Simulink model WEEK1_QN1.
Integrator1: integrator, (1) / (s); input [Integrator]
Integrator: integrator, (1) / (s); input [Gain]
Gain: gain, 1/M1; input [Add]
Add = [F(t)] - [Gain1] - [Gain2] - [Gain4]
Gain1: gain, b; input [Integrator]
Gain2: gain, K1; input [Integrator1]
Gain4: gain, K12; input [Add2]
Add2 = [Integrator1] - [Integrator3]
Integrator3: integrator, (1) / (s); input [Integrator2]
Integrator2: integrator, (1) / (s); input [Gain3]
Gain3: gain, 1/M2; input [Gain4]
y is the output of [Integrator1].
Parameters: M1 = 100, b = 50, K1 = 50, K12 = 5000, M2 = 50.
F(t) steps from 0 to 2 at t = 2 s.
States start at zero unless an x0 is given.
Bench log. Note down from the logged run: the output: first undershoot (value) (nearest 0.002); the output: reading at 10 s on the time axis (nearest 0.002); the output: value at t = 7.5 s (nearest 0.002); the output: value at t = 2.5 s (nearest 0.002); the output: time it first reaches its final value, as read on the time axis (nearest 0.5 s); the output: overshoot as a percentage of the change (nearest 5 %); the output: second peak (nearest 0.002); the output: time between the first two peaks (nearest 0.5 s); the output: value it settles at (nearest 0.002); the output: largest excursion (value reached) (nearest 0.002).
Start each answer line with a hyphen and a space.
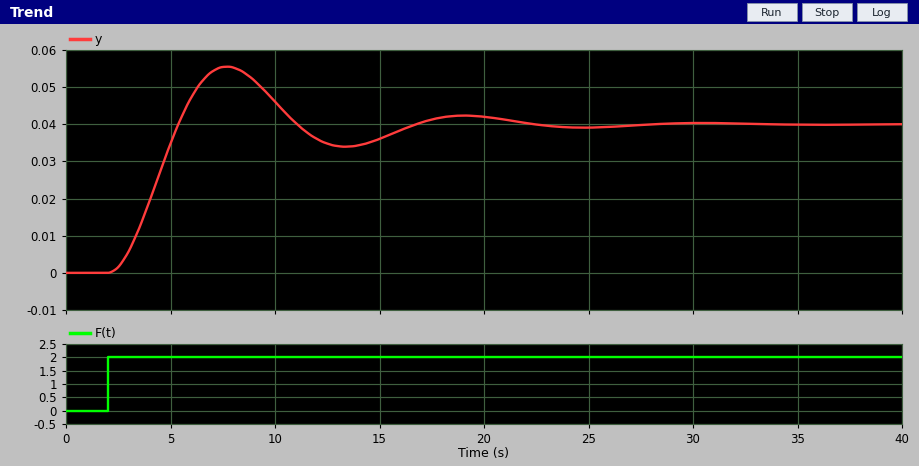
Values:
- 0.034
- 0.046
- 0.056
- 0.002
- 5.5 s
- 40 %
- 0.042
- 11.5 s
- 0.040
- 0.056
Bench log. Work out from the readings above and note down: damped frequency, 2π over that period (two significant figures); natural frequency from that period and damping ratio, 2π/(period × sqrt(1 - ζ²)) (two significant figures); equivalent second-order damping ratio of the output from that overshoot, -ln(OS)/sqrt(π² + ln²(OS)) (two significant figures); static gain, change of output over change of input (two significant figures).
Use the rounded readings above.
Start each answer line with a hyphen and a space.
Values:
- 0.55 rad/s
- 0.57 rad/s
- 0.28
- 0.020
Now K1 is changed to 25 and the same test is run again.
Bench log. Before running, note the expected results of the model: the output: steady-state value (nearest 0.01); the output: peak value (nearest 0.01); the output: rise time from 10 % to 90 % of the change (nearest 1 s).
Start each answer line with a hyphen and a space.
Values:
- 0.08
- 0.10
- 4 s
